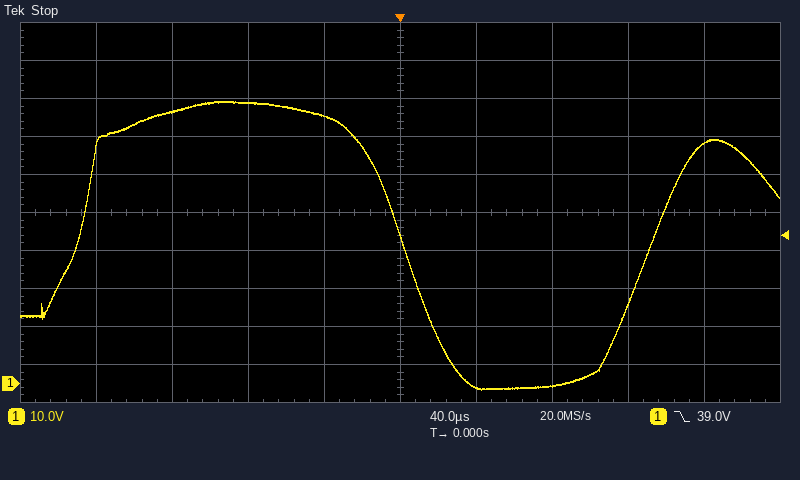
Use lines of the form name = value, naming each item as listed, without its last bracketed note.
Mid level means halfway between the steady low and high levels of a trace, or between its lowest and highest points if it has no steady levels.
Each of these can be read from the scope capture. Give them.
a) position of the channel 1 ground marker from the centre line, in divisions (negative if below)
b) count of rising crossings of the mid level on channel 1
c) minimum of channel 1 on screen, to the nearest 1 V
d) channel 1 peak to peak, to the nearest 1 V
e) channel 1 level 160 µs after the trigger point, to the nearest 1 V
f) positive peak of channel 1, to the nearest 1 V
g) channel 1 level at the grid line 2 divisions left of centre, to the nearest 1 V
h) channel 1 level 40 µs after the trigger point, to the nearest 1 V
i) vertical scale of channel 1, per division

position of the channel 1 ground marker from the centre line, in divisions = -4.5 div
count of rising crossings of the mid level on channel 1 = 2
minimum of channel 1 on screen, to the nearest 1 V = -2 V
channel 1 peak to peak, to the nearest 1 V = 76 V
channel 1 level 160 µs after the trigger point, to the nearest 1 V = 63 V
positive peak of channel 1, to the nearest 1 V = 74 V
channel 1 level at the grid line 2 divisions left of centre, to the nearest 1 V = 74 V
channel 1 level 40 µs after the trigger point, to the nearest 1 V = -1 V
vertical scale of channel 1, per division = 10 V
